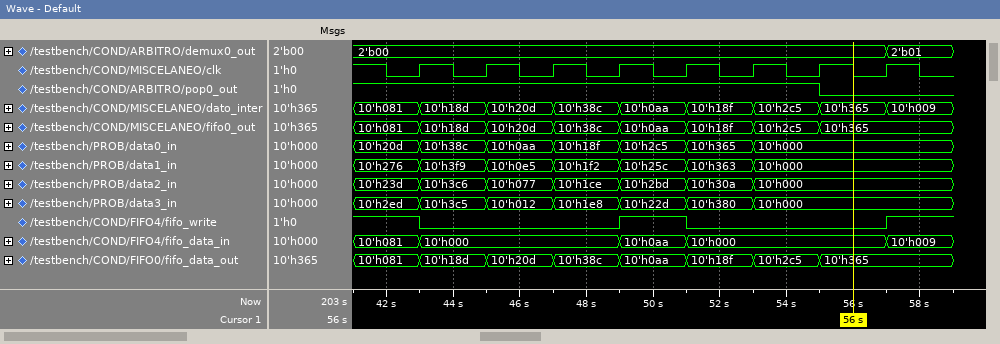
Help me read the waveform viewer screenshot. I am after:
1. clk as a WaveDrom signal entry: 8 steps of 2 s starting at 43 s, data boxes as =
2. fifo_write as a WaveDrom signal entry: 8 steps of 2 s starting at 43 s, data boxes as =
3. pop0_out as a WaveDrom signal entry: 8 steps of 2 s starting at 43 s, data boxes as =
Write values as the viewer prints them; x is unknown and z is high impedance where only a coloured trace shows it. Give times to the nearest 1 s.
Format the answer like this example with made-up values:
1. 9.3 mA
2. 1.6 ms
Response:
1. {name: 'clk', wave: 'p.......'}
2. {name: 'fifo_write', wave: '0..10..1'}
3. {name: 'pop0_out', wave: '1.....0.'}
